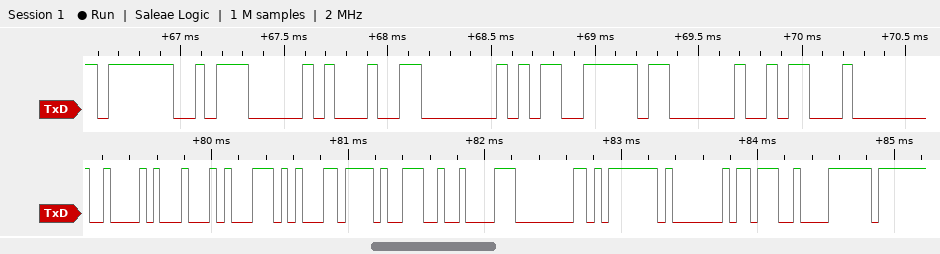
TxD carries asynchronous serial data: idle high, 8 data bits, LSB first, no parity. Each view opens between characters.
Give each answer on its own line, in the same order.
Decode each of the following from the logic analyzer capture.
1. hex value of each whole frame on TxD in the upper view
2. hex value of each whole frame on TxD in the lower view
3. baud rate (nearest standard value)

3F, 07, 91, 40, F3, 03, 1A
42, 44, 5C, EC, 39, C2, 80, FD, 01, 3B, F8
19200 baud
